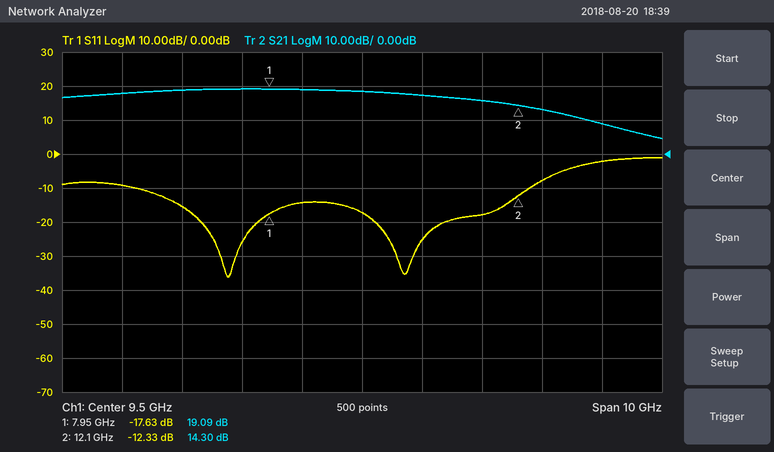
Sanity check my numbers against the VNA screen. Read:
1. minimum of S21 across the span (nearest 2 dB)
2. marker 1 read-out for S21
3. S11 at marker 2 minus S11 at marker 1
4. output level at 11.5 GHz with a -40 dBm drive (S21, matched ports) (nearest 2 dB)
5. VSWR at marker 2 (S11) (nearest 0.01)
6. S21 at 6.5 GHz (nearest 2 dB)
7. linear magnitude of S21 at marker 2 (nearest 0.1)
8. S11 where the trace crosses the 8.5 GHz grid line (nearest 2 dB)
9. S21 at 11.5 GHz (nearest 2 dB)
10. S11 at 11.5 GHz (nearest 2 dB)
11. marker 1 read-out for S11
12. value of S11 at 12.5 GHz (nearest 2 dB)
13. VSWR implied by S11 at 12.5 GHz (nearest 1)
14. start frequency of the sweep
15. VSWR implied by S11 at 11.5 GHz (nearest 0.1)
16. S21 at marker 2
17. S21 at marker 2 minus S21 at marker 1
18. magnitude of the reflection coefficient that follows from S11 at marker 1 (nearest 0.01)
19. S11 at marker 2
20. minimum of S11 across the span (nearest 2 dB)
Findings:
4 dB
19.09 dB
5.30 dB
-24 dBm
1.64
18 dB
5.2
-14 dB
16 dB
-18 dB
-17.63 dB
-8 dB
2
4.5 GHz
1.3
14.30 dB
-4.79 dB
0.13
-12.33 dB
-36 dB
